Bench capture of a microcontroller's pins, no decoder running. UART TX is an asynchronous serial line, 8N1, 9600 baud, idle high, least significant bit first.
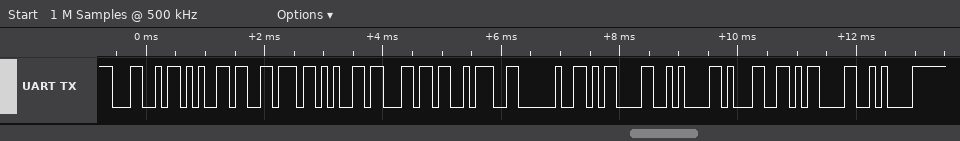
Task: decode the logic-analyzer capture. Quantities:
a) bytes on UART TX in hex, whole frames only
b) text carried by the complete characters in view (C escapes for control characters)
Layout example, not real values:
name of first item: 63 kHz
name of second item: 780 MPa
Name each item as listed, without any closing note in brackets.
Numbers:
bytes on UART TX in hex, whole frames only: 0x4C 0x65 0x76 0x65 0x6C 0x3A 0x20 0x0D 0x0A 0x31 0x0D 0x0A
text carried by the complete characters in view: "Level: \r\n1\r\n"
